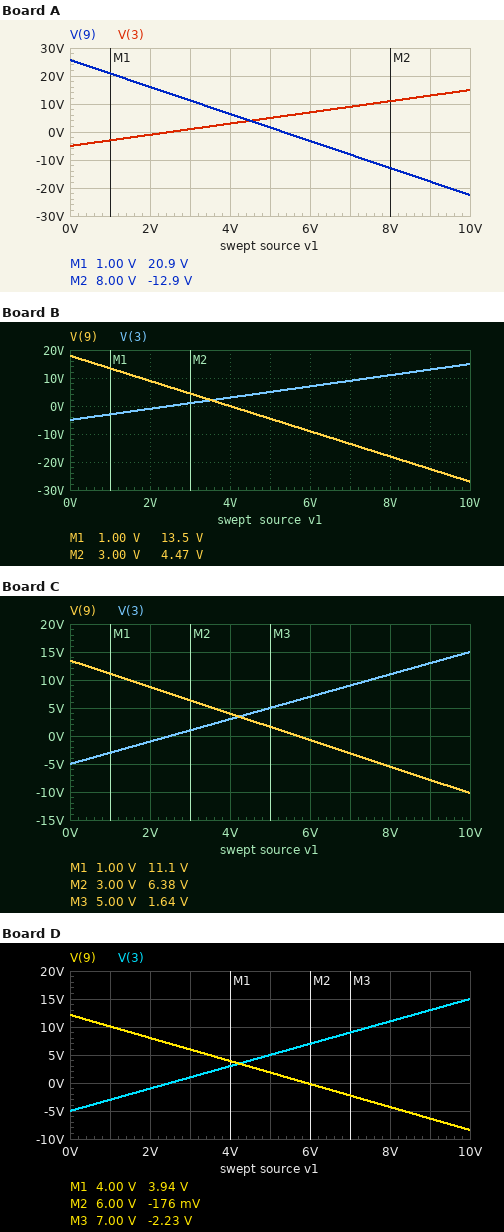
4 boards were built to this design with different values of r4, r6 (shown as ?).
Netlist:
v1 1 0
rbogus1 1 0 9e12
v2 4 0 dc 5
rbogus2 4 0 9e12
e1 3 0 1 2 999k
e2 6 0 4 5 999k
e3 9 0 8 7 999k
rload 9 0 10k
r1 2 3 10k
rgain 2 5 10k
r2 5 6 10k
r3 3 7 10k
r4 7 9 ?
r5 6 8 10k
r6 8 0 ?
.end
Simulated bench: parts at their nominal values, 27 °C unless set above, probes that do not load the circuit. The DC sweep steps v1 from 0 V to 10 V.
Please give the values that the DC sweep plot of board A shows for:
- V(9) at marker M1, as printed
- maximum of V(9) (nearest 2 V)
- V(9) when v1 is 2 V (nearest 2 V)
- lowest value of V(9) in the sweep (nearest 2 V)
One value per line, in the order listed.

20.9 V
26 V
16 V
-22 V
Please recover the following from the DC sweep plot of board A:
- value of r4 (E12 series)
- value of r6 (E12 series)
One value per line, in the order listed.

15 kΩ
27 kΩ
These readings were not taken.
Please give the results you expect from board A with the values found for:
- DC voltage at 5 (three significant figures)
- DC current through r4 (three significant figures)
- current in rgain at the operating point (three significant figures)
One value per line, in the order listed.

5.00 V
1.23 mA
500 µA
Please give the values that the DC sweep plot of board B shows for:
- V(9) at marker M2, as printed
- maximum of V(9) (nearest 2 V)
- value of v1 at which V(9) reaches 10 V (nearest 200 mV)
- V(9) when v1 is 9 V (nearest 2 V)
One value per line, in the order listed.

4.47 V
18 V
1.8 V
-22 V
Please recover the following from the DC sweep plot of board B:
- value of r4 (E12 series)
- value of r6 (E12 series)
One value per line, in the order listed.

18 kΩ
4.7 kΩ
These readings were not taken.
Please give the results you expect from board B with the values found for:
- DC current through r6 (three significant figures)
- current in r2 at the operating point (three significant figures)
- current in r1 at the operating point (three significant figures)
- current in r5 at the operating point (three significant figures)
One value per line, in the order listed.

680 µA
500 µA
500 µA
680 µA
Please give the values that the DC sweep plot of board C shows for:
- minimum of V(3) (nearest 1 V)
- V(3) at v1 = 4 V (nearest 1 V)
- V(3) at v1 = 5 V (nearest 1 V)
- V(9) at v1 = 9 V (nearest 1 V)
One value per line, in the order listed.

-5 V
3 V
5 V
-8 V
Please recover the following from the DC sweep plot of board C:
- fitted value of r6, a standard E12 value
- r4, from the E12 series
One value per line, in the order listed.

15 kΩ
6.8 kΩ
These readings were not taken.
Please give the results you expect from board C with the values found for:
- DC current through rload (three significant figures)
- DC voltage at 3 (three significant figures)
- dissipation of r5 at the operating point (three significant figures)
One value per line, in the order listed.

1.35 mA
-5.00 V
1.60 mW
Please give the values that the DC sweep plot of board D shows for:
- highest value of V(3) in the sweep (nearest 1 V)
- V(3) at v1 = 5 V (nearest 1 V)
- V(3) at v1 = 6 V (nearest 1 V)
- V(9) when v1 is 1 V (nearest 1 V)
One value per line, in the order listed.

15 V
5 V
7 V
10 V
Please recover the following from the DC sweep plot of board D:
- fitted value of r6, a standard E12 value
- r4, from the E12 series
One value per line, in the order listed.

15 kΩ
5.6 kΩ
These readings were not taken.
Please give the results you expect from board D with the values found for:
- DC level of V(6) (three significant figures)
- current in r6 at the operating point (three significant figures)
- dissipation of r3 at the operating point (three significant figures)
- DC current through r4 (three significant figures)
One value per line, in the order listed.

10.0 V
400 µA
12.1 mW
1.10 mA
